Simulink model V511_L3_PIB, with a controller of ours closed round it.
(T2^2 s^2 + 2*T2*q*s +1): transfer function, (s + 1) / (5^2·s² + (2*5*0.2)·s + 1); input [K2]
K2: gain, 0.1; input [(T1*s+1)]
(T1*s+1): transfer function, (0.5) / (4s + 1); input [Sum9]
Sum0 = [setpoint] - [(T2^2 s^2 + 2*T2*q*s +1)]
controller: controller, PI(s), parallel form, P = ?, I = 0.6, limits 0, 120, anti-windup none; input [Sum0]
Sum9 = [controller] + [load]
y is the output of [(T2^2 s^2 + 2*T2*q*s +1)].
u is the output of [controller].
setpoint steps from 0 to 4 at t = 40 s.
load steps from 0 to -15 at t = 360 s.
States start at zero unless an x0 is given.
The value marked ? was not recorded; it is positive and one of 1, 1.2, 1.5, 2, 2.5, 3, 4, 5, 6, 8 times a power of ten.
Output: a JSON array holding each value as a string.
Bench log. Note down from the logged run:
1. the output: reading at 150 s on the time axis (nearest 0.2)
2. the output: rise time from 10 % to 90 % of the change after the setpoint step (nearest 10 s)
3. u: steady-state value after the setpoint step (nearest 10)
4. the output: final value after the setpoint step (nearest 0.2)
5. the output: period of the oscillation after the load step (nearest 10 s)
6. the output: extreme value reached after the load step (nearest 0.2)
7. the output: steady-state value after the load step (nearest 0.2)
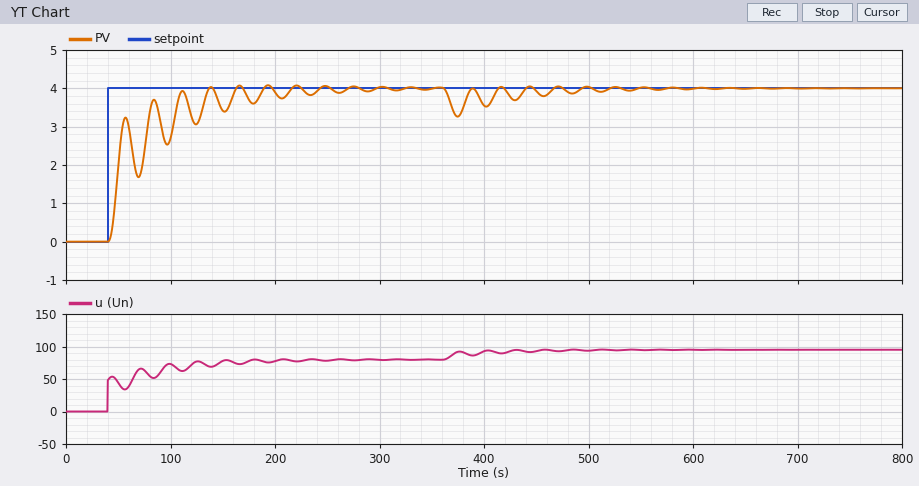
["3.4", "40 s", "80", "4.0", "30 s", "3.2", "4.0"]
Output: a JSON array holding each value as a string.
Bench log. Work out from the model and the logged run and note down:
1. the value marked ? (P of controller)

["12"]
